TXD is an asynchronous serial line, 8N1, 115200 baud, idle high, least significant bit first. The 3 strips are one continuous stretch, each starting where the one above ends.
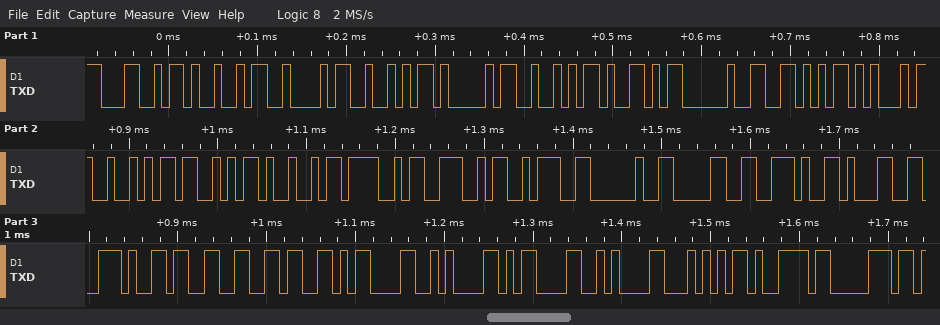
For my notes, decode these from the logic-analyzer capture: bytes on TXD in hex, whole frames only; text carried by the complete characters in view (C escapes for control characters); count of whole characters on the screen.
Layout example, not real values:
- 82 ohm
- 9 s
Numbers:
- 4C 49 42 52 41 52 59 20 56 45 52 53 49 4F 4E 3A 20 30 2E 31 2E 33 36 0D 0A 0D 0A 54 79 70
- "LIBRARY VERSION: 0.1.36\r\n\r\nTyp"
- 30
